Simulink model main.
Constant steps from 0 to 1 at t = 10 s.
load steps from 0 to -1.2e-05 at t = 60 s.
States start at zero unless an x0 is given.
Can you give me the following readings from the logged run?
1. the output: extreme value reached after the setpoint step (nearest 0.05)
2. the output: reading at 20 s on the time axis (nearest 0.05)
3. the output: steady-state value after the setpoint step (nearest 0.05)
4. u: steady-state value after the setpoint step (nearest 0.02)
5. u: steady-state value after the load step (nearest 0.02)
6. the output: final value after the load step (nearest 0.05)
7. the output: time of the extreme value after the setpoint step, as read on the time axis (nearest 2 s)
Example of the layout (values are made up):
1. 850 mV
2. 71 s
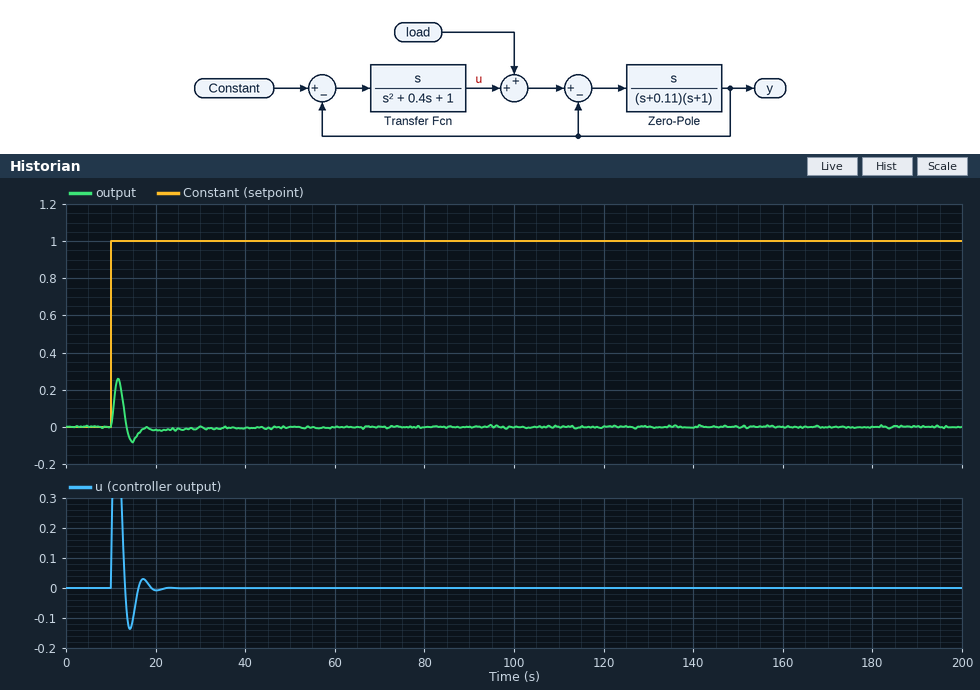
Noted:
1. 0.25
2. 0.00
3. 0.00
4. 0.00
5. 0.00
6. 0.00
7. 12 s
